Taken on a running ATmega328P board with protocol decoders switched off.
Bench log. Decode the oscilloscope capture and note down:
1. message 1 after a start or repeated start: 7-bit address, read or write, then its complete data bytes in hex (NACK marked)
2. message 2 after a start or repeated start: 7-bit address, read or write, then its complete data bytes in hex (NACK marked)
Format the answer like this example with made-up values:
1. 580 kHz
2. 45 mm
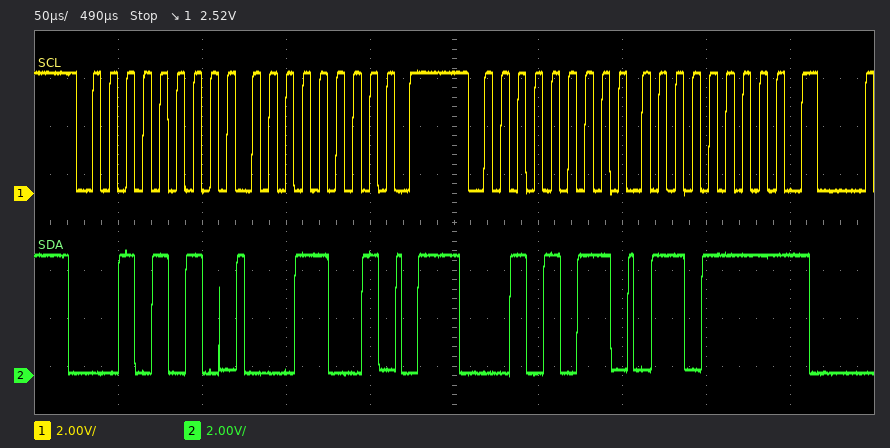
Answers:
1. 0x15 write: 19
2. 0x15 read: 6F NACK
